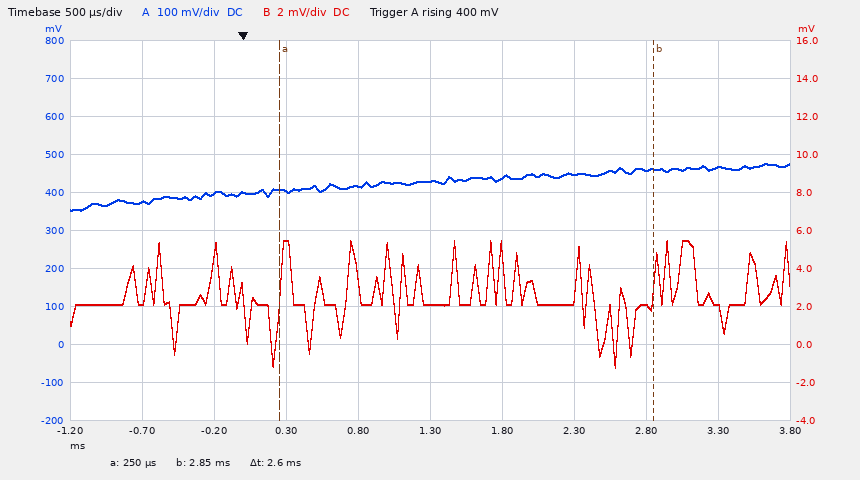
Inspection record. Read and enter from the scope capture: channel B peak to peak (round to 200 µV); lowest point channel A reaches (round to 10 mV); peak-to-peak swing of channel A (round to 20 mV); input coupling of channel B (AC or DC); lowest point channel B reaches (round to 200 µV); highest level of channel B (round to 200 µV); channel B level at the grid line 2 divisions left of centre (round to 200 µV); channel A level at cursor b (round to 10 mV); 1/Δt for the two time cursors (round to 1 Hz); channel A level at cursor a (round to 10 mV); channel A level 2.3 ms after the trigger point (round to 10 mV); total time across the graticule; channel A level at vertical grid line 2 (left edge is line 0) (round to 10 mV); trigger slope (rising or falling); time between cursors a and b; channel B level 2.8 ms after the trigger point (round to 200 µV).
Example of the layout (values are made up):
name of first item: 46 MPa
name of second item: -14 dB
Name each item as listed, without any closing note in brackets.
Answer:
channel B peak to peak: 6.6 mV
lowest point channel A reaches: 350 mV
peak-to-peak swing of channel A: 120 mV
input coupling of channel B: DC
lowest point channel B reaches: -1.2 mV
highest level of channel B: 5.4 mV
channel B level at the grid line 2 divisions left of centre: 5.2 mV
channel A level at cursor b: 460 mV
1/Δt for the two time cursors: 385 Hz
channel A level at cursor a: 410 mV
channel A level 2.3 ms after the trigger point: 450 mV
total time across the graticule: 5 ms
channel A level at vertical grid line 2 (left edge is line 0): 400 mV
trigger slope: rising
time between cursors a and b: 2.6 ms
channel B level 2.8 ms after the trigger point: 2.0 mV
